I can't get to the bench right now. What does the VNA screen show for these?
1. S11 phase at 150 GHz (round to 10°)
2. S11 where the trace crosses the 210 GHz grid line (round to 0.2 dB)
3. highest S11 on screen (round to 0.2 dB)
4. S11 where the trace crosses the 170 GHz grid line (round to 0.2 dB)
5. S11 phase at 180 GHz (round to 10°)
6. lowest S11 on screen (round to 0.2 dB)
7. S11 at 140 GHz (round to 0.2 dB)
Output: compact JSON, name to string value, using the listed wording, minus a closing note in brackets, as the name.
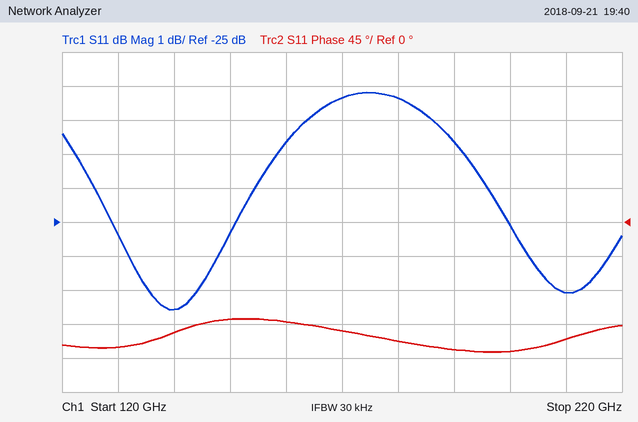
{"S11 phase at 150 GHz": "-130°", "S11 where the trace crosses the 210 GHz grid line": "-27.0 dB", "highest S11 on screen": "-21.2 dB", "S11 where the trace crosses the 170 GHz grid line": "-21.4 dB", "S11 phase at 180 GHz": "-160°", "lowest S11 on screen": "-27.6 dB", "S11 at 140 GHz": "-27.6 dB"}
